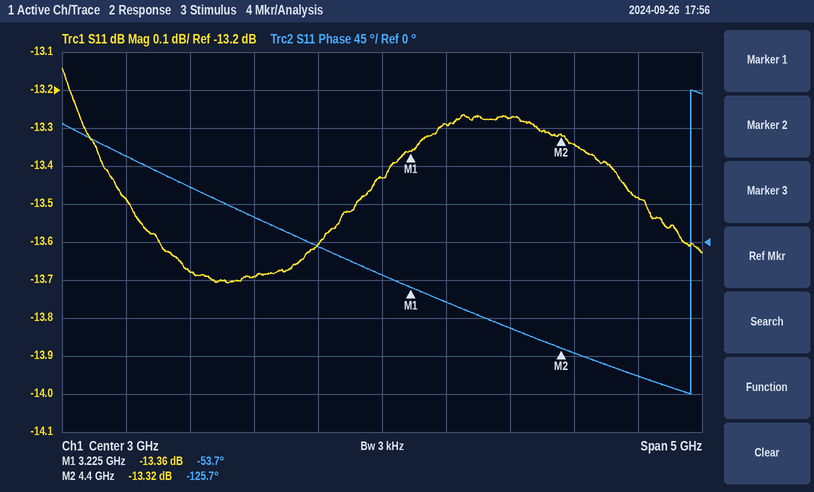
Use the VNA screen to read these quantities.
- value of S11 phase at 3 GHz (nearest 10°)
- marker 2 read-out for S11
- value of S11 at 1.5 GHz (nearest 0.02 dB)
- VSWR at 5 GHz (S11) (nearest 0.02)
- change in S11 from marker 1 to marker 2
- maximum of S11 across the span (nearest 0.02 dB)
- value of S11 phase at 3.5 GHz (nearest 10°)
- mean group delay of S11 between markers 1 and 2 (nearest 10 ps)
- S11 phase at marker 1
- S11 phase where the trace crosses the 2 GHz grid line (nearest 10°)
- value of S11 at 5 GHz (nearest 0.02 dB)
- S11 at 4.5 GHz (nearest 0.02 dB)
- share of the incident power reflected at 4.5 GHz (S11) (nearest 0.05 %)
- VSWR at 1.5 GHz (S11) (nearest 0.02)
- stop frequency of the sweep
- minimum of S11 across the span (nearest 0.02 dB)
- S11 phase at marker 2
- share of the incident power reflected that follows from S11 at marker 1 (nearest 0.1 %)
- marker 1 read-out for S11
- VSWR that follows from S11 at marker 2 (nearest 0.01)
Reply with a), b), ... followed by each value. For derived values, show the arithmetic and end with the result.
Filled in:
a) -40°
b) -13.32 dB
c) -13.68 dB
d) |Γ| = 10^(-13.48/20) = 0.2118; VSWR = (1 + 0.2118)/(1 − 0.2118) ≈ 1.54
e) -13.32 − (-13.36) = 0.04 dB
f) -13.14 dB
g) -70°
h) −(-125.7° − (-53.7°))/(360° × 1.175 GHz) ≈ 170 ps
i) -53.7°
j) 30°
k) -13.48 dB
l) -13.34 dB
m) 10^(-13.34/10) ≈ 4.63 %, so 4.65 % to the nearest 0.05 %
n) |Γ| = 10^(-13.68/20) = 0.2070; VSWR = (1 + 0.2070)/(1 − 0.2070) ≈ 1.52
o) 5.5 GHz
p) -13.70 dB
q) -125.7°
r) 10^(-13.36/10) ≈ 4.6 %
s) -13.36 dB
t) (1 + 0.2158)/(1 − 0.2158) ≈ 1.55
